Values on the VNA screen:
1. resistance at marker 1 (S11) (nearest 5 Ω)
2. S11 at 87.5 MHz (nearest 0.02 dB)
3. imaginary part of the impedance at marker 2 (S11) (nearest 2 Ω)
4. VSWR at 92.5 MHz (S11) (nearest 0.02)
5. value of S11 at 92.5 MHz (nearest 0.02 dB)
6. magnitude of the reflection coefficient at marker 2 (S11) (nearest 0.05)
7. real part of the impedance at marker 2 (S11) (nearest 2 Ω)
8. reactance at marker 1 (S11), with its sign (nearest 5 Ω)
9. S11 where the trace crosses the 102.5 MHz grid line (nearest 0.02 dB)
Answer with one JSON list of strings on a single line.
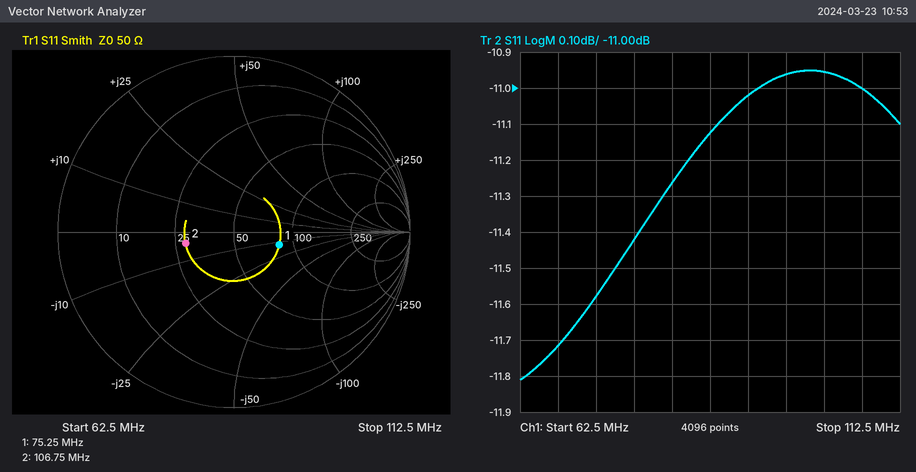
["85 Ω", "-11.12 dB", "-4 Ω", "1.78", "-11.02 dB", "0.30", "28 Ω", "-15 Ω", "-10.96 dB"]
